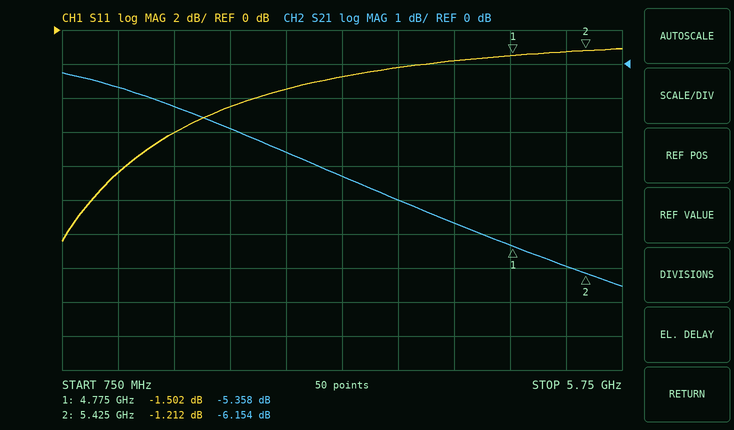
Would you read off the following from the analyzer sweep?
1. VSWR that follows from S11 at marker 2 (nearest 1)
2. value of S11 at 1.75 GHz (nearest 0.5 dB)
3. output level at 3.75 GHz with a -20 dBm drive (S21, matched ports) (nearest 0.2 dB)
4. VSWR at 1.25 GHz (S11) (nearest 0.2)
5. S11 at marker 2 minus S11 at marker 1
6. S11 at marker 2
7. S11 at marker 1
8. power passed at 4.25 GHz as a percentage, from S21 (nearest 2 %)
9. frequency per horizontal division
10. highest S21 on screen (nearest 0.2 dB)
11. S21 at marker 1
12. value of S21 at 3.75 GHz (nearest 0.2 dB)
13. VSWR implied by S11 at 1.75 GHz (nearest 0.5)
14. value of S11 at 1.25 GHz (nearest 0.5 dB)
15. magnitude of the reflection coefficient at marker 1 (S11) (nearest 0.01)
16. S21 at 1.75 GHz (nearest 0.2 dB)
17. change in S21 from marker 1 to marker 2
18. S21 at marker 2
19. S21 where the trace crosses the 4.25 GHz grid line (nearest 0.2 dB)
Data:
14
-6.0 dB
-24.0 dBm
2.2
0.290 dB
-1.212 dB
-1.502 dB
34 %
500 MHz
-0.2 dB
-5.358 dB
-4.0 dB
3.0
-8.5 dB
0.84
-1.2 dB
-0.796 dB
-6.154 dB
-4.6 dB
